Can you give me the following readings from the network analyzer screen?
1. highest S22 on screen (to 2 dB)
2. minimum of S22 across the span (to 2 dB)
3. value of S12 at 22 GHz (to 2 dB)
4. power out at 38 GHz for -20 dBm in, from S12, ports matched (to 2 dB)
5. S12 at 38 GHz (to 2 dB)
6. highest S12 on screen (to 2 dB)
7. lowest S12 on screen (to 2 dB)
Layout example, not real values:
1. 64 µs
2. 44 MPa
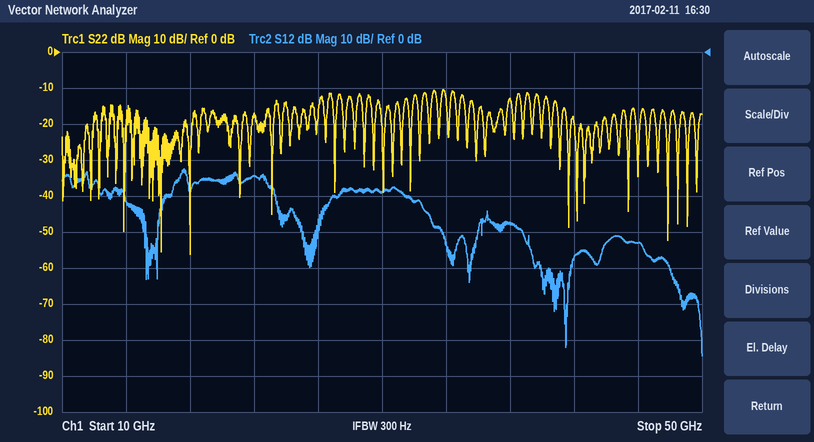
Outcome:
1. -10 dB
2. -56 dB
3. -34 dB
4. -68 dBm
5. -48 dB
6. -32 dB
7. -84 dB
